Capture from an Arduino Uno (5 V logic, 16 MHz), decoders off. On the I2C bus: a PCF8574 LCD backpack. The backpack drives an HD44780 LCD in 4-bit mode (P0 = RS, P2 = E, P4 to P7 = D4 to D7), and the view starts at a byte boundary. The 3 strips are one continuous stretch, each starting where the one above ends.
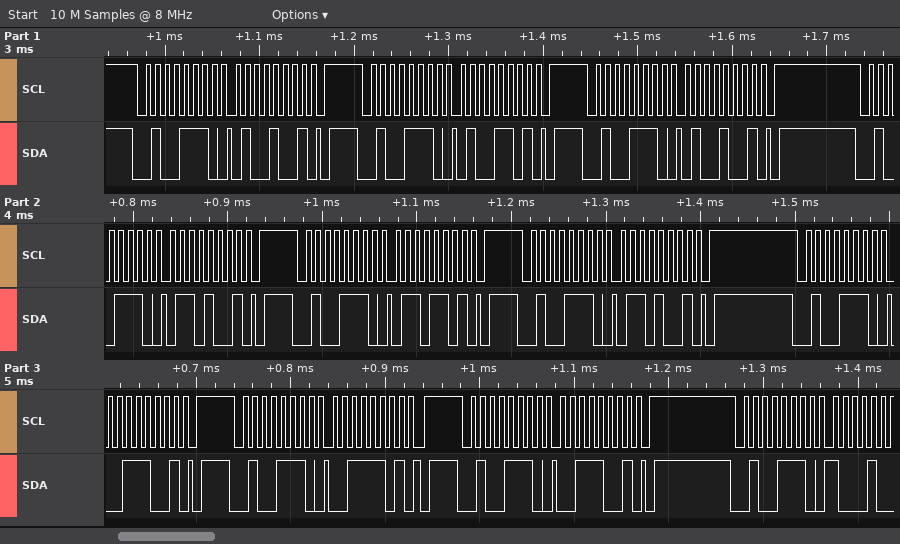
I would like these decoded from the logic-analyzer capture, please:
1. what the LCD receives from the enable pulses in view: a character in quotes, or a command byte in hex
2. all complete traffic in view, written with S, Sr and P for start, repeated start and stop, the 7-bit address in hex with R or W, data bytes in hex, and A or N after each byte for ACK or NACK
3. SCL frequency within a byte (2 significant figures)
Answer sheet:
'F'
S 27W A 49 A P S 27W A 4D A P S 27W A 49 A P S 27W A 69 A P S 27W A 6D A P S 27W A 69 A P S 27W A 39 A P S 27W A 3D A P S 27W A 39 A P S 27W A
100 kHz
